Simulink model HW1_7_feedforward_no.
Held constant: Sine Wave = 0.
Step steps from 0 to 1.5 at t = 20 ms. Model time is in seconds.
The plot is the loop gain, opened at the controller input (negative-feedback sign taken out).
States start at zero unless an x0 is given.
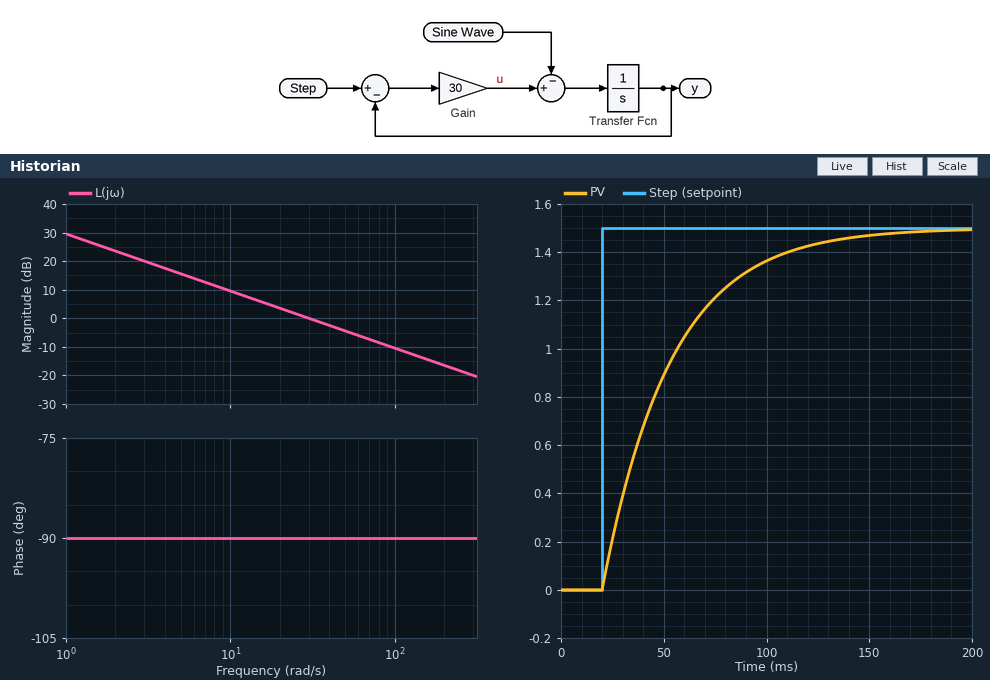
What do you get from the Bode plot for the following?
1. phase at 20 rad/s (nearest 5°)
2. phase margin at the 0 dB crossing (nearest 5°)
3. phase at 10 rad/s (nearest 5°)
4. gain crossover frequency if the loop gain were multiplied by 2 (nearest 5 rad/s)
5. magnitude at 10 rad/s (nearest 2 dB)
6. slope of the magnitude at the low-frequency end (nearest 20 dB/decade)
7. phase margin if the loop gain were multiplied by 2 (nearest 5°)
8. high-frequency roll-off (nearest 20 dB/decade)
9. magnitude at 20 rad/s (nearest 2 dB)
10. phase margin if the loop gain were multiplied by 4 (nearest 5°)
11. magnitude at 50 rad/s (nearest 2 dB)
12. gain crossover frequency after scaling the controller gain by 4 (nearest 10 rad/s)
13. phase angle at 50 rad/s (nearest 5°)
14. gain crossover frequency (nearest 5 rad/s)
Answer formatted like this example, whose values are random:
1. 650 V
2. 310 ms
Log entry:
1. -90°
2. 90°
3. -90°
4. 60 rad/s
5. 10 dB
6. -20 dB/decade
7. 90°
8. -20 dB/decade
9. 4 dB
10. 90°
11. -4 dB
12. 120 rad/s
13. -90°
14. 30 rad/s
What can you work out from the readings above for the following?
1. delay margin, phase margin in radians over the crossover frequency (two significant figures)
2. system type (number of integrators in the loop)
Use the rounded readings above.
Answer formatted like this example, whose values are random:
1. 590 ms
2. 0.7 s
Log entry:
1. 0.052 s
2. 1
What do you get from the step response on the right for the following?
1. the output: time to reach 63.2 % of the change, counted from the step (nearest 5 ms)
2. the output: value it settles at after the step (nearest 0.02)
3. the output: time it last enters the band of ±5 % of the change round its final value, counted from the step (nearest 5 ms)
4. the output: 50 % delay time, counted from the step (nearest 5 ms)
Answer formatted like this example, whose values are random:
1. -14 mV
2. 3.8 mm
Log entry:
1. 35 ms
2. 1.50
3. 100 ms
4. 25 ms
